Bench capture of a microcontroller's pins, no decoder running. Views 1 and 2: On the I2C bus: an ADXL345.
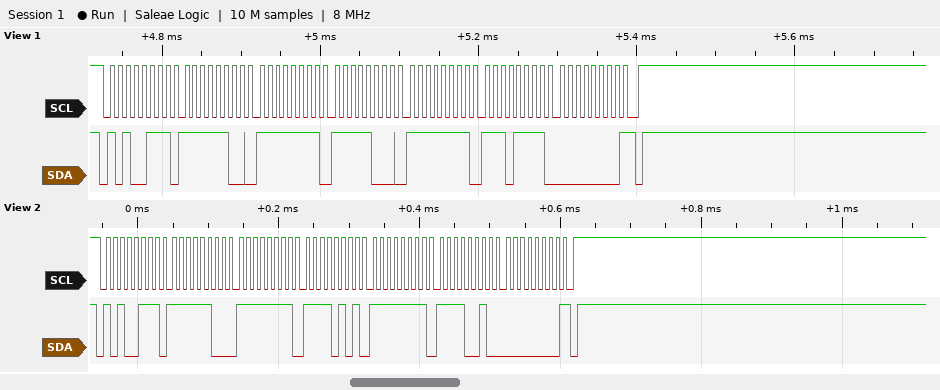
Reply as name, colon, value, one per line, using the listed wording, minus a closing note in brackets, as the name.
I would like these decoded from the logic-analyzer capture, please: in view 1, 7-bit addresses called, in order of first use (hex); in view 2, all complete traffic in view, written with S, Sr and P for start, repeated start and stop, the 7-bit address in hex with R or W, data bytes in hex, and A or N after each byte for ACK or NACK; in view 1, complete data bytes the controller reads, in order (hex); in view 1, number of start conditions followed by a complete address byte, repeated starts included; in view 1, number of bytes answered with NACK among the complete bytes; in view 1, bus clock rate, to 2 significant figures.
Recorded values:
in view 1, 7-bit addresses called, in order of first use: 0x53
in view 2, all complete traffic in view, written with S, Sr and P for start, repeated start and stop, the 7-bit address in hex with R or W, data bytes in hex, and A or N after each byte for ACK or NACK: S 53R A FC A FF A F5 A FF A F2 A 00 N P
in view 1, complete data bytes the controller reads, in order: FC FF F8 FF EF 00
in view 1, number of start conditions followed by a complete address byte, repeated starts included: 1
in view 1, number of bytes answered with NACK among the complete bytes: 1
in view 1, bus clock rate, to 2 significant figures: 100 kHz
